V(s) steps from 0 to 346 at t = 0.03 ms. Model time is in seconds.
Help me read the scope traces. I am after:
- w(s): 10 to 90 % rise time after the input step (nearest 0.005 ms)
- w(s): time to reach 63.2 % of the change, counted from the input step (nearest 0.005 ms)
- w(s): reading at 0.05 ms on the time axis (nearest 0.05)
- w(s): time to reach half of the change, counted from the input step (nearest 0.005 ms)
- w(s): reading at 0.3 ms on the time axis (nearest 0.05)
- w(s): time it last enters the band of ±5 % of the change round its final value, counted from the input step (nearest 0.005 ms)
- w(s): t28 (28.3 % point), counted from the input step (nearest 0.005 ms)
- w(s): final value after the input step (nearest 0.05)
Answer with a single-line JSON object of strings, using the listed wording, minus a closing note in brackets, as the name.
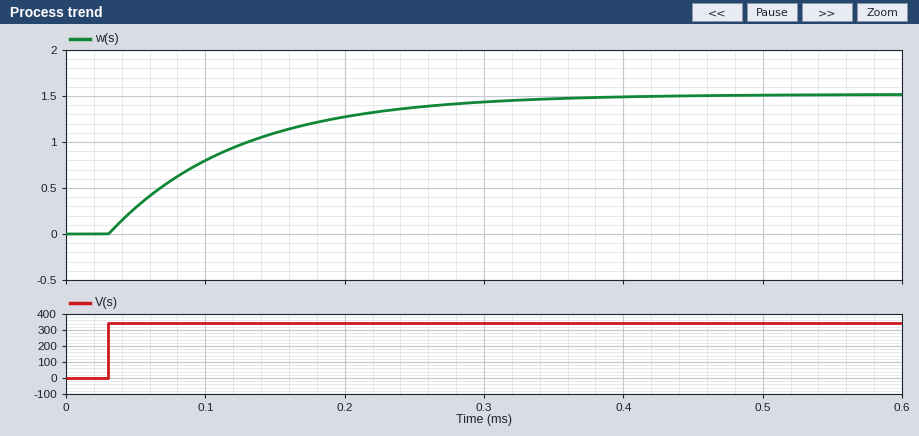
{"w(s): 10 to 90 % rise time after the input step": "0.205 ms", "w(s): time to reach 63.2 % of the change, counted from the input step": "0.095 ms", "w(s): reading at 0.05 ms on the time axis": "0.30", "w(s): time to reach half of the change, counted from the input step": "0.065 ms", "w(s): reading at 0.3 ms on the time axis": "1.45", "w(s): time it last enters the band of ±5 % of the change round its final value, counted from the input step": "0.280 ms", "w(s): t28 (28.3 % point), counted from the input step": "0.030 ms", "w(s): final value after the input step": "1.50"}
